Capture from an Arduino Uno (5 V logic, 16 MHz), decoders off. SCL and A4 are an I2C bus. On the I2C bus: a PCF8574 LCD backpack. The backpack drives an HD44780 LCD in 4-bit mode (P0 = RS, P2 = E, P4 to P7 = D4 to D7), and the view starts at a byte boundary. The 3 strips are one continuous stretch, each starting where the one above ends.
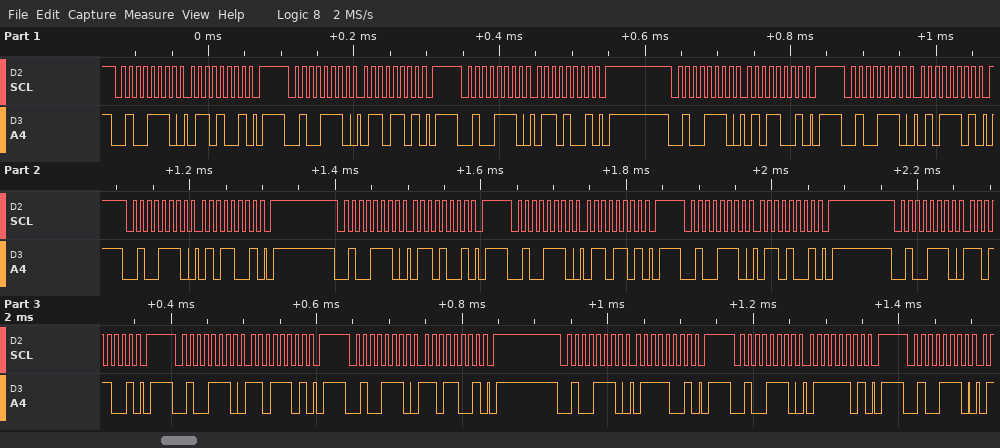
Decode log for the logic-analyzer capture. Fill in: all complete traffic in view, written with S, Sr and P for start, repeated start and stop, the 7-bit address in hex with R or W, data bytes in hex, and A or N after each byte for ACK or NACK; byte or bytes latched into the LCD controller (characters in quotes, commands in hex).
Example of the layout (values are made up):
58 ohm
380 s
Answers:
S 27W A 69 A P S 27W A 6D A P S 27W A 69 A P S 27W A 59 A P S 27W A 5D A P S 27W A 59 A P S 27W A 69 A P S 27W A 6D A P S 27W A 69 A P S 27W A D9 A P S 27W A DD A P S 27W A D9 A P S 27W A 79 A P S 27W A 7D A P S 27W A
'e' 'm'
